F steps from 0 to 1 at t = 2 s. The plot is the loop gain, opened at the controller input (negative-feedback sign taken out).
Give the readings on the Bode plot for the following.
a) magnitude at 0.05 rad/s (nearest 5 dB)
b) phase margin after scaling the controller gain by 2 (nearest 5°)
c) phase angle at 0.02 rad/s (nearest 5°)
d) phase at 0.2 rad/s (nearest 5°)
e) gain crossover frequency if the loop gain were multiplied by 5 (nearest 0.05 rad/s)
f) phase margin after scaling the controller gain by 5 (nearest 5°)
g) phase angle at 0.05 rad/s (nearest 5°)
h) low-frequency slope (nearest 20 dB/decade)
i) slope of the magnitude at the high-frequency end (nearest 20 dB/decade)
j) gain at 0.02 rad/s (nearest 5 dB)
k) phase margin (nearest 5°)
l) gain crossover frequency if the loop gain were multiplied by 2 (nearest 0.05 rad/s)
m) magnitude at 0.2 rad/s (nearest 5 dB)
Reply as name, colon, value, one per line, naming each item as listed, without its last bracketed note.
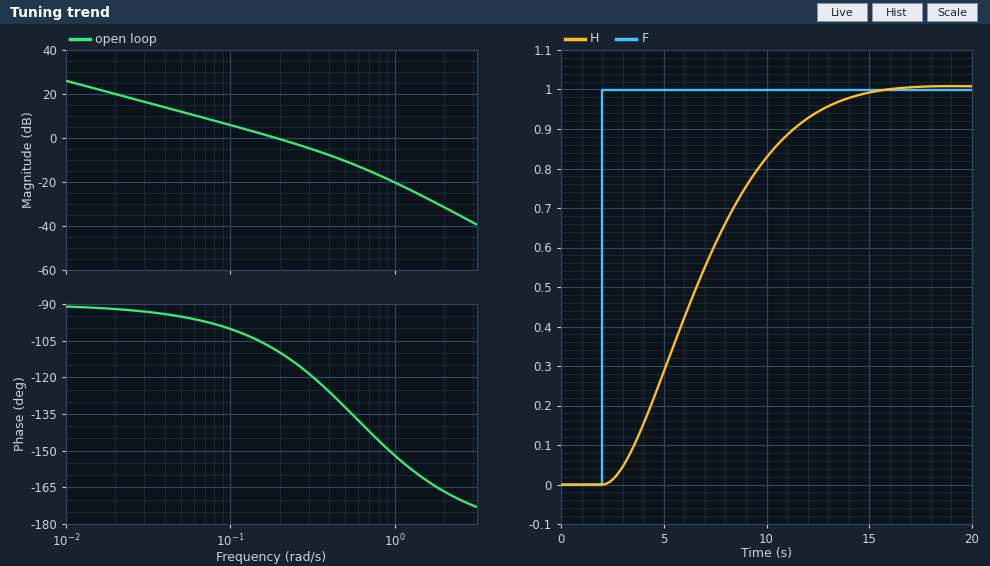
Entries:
magnitude at 0.05 rad/s: 10 dB
phase margin after scaling the controller gain by 2: 60°
phase angle at 0.02 rad/s: -90°
phase at 0.2 rad/s: -110°
gain crossover frequency if the loop gain were multiplied by 5: 0.65 rad/s
phase margin after scaling the controller gain by 5: 40°
phase angle at 0.05 rad/s: -95°
low-frequency slope: -20 dB/decade
slope of the magnitude at the high-frequency end: -40 dB/decade
gain at 0.02 rad/s: 20 dB
phase margin: 70°
gain crossover frequency if the loop gain were multiplied by 2: 0.35 rad/s
magnitude at 0.2 rad/s: 0 dB
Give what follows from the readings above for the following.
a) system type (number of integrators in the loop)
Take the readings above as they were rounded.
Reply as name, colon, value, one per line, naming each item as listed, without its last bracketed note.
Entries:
system type: 1
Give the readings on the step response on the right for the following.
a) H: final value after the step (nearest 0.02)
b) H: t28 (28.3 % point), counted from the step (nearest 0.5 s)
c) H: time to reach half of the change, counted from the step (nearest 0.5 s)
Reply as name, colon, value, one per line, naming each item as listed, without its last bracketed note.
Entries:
H: final value after the step: 1.00
H: t28 (28.3 % point), counted from the step: 3.0 s
H: time to reach half of the change, counted from the step: 4.5 s
